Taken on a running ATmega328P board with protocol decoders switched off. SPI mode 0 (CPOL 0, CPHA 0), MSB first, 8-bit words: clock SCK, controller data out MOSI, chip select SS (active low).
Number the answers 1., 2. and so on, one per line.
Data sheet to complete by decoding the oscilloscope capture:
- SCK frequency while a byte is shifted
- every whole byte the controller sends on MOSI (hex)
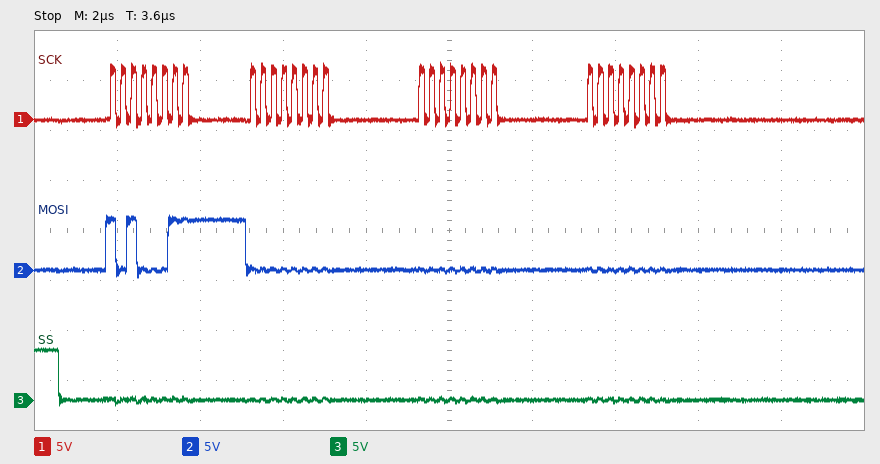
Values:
1. 4 MHz
2. A3 00 00 00
